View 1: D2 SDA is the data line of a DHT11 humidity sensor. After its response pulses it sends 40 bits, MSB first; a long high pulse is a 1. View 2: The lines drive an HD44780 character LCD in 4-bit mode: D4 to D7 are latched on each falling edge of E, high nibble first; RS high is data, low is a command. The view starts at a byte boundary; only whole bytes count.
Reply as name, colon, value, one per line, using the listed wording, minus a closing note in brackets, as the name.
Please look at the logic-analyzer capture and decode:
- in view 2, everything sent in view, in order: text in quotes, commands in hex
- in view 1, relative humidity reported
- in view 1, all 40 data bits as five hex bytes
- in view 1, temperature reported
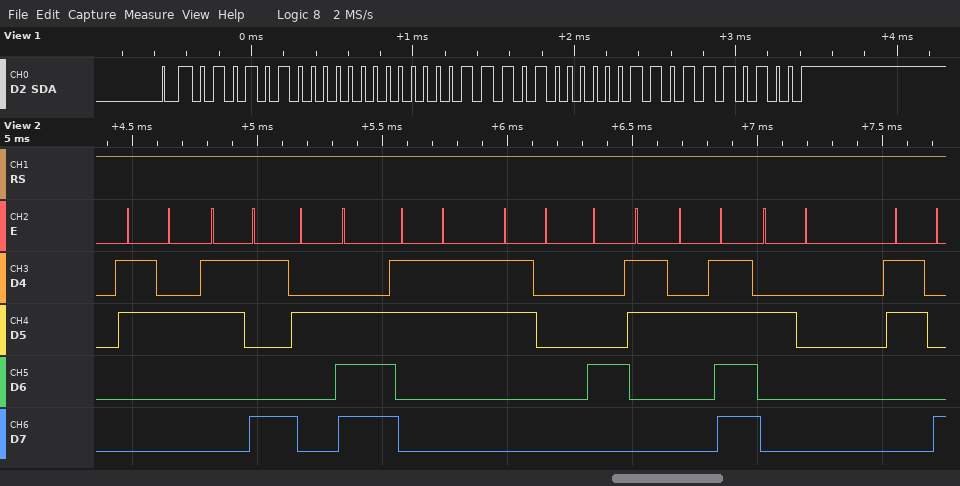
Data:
in view 2, everything sent in view, in order: text in quotes, commands in hex: "29.30C/ 8"
in view 1, relative humidity reported: 84 %
in view 1, all 40 data bits as five hex bytes: 54 00 1D 03 74
in view 1, temperature reported: 29.3 °C
